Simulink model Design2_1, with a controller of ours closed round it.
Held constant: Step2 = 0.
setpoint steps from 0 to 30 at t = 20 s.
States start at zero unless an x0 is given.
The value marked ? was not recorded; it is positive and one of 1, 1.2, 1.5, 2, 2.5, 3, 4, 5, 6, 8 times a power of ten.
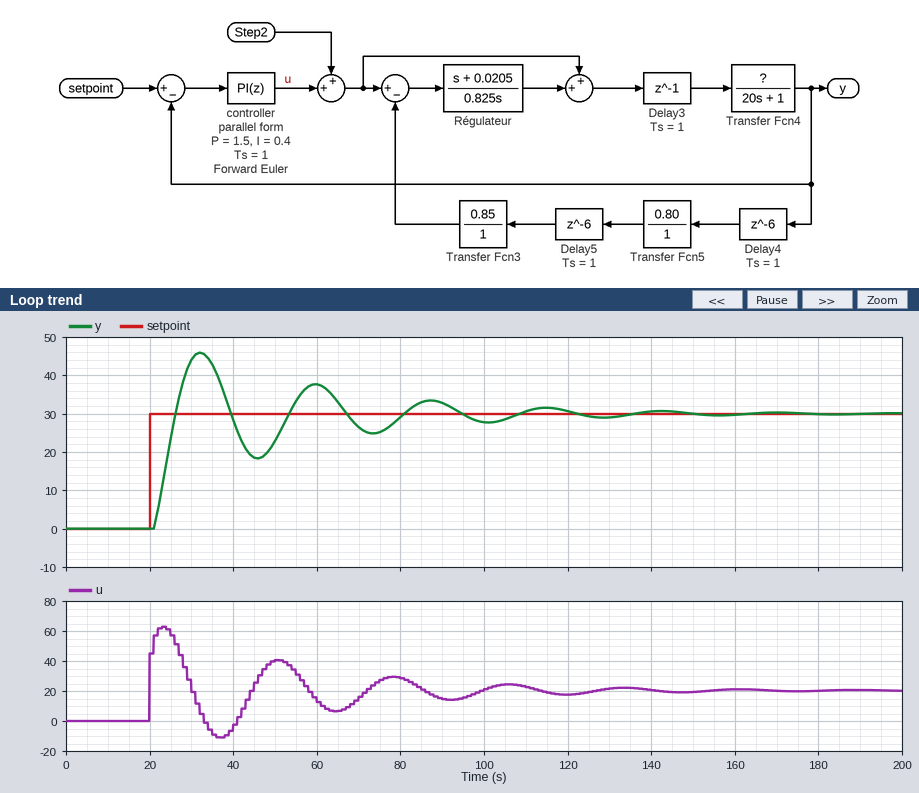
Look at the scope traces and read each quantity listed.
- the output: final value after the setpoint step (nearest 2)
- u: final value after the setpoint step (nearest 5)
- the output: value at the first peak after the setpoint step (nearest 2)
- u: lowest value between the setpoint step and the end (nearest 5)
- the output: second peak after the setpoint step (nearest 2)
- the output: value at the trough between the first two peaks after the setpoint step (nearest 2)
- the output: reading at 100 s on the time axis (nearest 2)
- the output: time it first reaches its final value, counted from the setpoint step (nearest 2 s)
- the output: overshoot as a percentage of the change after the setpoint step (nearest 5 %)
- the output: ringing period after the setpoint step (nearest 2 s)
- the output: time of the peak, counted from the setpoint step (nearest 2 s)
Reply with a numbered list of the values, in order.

1. 30
2. 20
3. 46
4. -10
5. 38
6. 18
7. 28
8. 6 s
9. 55 %
10. 28 s
11. 12 s
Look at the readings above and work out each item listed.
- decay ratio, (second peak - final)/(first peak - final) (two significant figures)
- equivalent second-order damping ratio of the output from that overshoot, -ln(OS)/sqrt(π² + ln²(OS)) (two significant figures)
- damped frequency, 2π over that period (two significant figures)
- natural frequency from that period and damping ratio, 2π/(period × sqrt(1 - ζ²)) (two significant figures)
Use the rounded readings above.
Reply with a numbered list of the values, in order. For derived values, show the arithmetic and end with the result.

1. (38 - 30) / (46 - 30) = 0.50
2. ln(0.55) = -0.598; 0.598 / sqrt(9.870 + 0.357) = 0.19
3. 2π / 28 = 0.22 rad/s
4. 2π / (28 × sqrt(1 - 0.19²)) = 0.23 rad/s
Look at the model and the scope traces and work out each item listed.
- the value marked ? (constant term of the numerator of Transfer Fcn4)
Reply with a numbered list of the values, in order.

1. 1
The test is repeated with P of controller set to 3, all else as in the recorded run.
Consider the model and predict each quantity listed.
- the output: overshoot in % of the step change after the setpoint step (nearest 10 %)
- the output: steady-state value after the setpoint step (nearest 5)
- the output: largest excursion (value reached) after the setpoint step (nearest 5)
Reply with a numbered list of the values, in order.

1. 30 %
2. 30
3. 40
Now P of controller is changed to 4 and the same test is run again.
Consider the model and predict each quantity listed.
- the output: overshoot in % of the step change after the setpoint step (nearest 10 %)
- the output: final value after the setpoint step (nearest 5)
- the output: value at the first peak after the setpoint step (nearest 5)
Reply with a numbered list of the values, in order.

1. 30 %
2. 30
3. 40
